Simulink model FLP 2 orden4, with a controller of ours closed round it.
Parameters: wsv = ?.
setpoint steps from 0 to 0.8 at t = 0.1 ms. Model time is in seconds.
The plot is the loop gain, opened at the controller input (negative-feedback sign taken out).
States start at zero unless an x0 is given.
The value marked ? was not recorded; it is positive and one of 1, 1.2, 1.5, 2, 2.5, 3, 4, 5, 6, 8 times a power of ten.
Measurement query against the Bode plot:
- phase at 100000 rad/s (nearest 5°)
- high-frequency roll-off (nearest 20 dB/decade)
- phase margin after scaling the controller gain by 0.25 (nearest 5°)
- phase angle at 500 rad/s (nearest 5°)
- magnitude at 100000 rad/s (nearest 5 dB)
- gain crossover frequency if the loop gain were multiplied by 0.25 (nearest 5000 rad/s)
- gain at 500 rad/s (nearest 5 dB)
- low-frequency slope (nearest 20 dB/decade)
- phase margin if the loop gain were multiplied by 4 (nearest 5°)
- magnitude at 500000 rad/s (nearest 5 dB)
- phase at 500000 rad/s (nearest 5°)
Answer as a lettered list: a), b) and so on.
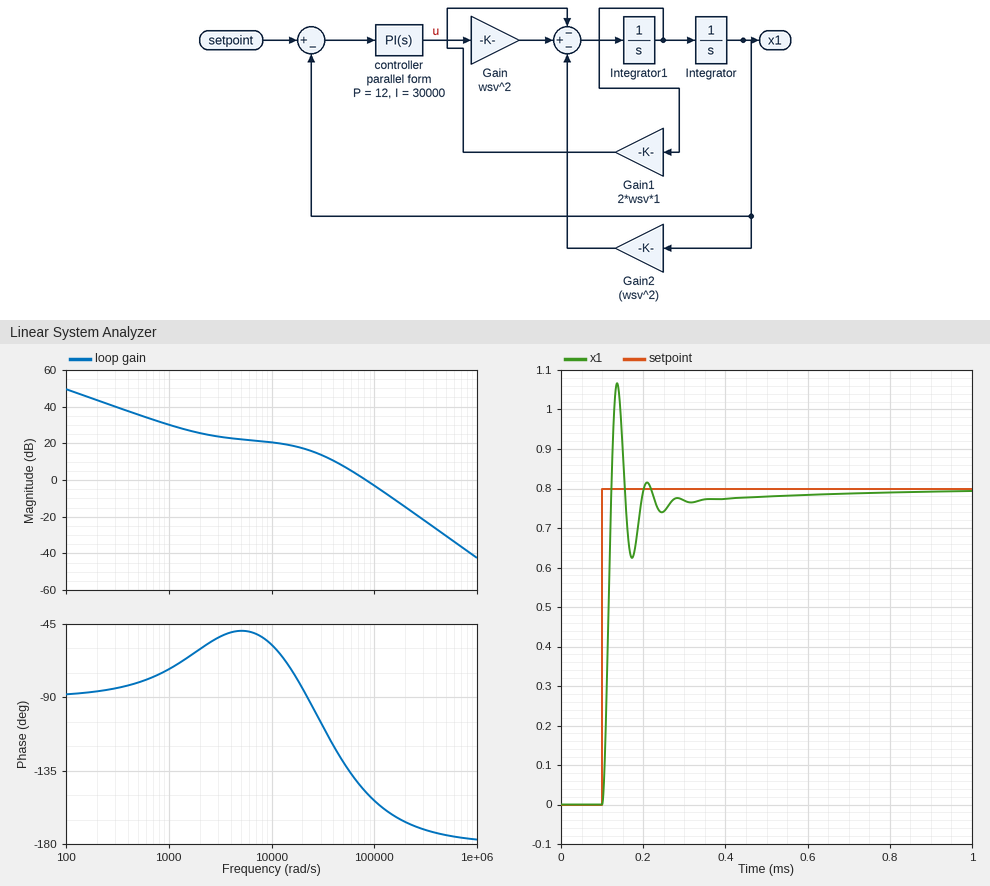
a) -155°
b) -40 dB/decade
c) 65°
d) -80°
e) -5 dB
f) 35000 rad/s
g) 35 dB
h) -20 dB/decade
i) 15°
j) -30 dB
k) -175°
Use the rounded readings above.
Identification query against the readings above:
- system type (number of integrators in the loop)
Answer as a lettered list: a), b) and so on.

a) 1
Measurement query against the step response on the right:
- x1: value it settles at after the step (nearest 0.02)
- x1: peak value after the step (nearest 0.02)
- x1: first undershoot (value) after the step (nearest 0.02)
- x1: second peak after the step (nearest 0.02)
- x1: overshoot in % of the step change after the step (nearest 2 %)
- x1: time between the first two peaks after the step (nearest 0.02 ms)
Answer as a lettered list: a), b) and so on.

a) 0.80
b) 1.06
c) 0.62
d) 0.82
e) 34 %
f) 0.08 ms
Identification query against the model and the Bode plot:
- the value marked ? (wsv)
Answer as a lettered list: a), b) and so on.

a) 25000
